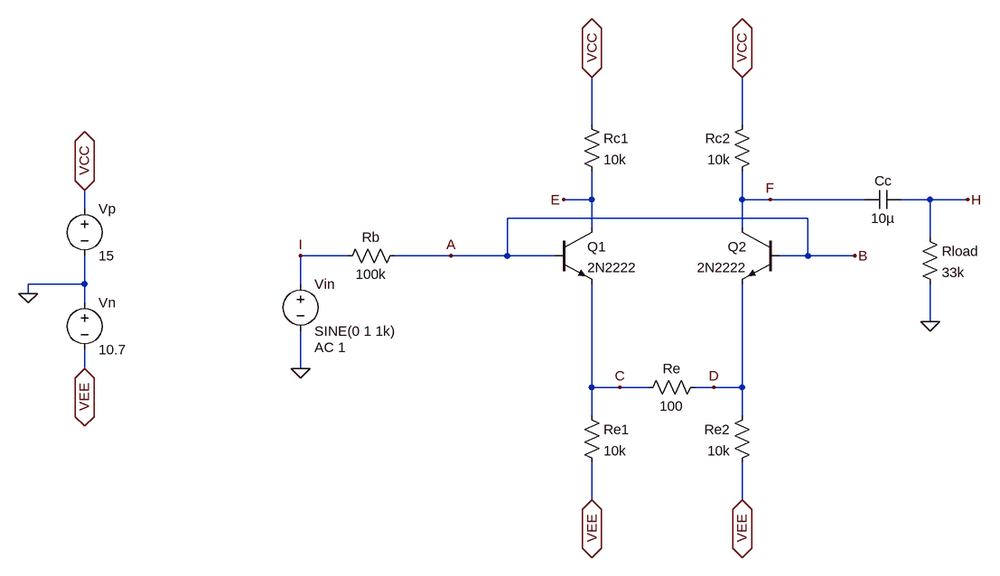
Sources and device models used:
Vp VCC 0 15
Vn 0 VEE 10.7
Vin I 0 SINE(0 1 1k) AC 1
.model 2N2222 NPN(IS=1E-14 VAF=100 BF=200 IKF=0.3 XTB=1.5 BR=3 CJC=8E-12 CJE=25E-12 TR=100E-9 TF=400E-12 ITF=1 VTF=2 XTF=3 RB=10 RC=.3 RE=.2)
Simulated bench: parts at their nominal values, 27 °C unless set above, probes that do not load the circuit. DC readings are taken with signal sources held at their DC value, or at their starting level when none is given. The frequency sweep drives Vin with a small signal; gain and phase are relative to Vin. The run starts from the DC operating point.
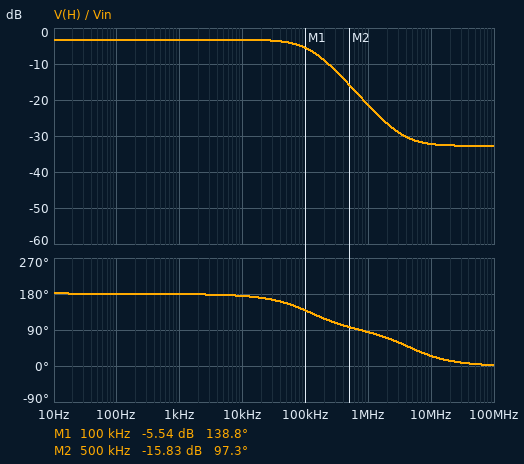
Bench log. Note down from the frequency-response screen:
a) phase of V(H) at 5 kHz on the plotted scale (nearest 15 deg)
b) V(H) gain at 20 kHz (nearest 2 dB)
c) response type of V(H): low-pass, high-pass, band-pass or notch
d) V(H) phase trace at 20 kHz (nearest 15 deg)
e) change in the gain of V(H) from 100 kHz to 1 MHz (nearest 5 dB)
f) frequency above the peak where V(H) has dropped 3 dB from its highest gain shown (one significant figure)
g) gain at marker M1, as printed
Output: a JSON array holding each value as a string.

["180 deg", "-4 dB", "low-pass", "165 deg", "-15 dB", "100 kHz", "-5.54 dB"]
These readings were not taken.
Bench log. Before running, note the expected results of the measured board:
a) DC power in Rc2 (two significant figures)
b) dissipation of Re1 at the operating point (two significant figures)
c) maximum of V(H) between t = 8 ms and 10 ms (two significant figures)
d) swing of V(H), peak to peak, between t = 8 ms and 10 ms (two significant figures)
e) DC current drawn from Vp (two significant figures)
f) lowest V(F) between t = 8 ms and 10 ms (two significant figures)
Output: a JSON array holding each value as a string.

["8.4 mW", "8.4 mW", "690 mV", "1.4 V", "1.8 mA", "5.2 V"]
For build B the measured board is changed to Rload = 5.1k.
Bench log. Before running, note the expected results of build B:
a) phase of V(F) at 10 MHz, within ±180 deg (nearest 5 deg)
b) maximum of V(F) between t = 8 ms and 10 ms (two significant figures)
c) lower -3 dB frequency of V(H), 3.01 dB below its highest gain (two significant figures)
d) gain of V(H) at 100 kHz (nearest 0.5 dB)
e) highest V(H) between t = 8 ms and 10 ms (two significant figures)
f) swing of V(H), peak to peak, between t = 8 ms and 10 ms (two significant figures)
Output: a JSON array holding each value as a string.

["35 deg", "6.2 V", "1.1 Hz", "-12.0 dB", "310 mV", "610 mV"]
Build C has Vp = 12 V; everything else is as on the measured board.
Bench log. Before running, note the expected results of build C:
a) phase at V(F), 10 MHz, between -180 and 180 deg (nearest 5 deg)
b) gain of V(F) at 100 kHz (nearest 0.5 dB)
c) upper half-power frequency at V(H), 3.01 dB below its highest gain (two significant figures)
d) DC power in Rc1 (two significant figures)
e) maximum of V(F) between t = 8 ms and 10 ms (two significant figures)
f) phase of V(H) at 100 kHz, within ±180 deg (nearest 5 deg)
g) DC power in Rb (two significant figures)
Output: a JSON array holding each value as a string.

["20 deg", "-6.0 dB", "100 kHz", "8.3 mW", "3.6 V", "135 deg", "7.8 µW"]
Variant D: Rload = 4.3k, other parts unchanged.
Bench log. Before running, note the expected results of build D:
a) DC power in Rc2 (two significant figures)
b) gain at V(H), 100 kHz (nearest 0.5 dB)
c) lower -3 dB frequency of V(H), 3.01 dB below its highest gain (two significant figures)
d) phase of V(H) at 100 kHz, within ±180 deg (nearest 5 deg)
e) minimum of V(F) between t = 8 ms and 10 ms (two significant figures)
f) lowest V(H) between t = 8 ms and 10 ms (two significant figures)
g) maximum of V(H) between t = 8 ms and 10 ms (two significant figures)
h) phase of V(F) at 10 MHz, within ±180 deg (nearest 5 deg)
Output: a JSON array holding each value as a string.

["8.4 mW", "-13.0 dB", "1.1 Hz", "145 deg", "5.6 V", "-270 mV", "270 mV", "35 deg"]
